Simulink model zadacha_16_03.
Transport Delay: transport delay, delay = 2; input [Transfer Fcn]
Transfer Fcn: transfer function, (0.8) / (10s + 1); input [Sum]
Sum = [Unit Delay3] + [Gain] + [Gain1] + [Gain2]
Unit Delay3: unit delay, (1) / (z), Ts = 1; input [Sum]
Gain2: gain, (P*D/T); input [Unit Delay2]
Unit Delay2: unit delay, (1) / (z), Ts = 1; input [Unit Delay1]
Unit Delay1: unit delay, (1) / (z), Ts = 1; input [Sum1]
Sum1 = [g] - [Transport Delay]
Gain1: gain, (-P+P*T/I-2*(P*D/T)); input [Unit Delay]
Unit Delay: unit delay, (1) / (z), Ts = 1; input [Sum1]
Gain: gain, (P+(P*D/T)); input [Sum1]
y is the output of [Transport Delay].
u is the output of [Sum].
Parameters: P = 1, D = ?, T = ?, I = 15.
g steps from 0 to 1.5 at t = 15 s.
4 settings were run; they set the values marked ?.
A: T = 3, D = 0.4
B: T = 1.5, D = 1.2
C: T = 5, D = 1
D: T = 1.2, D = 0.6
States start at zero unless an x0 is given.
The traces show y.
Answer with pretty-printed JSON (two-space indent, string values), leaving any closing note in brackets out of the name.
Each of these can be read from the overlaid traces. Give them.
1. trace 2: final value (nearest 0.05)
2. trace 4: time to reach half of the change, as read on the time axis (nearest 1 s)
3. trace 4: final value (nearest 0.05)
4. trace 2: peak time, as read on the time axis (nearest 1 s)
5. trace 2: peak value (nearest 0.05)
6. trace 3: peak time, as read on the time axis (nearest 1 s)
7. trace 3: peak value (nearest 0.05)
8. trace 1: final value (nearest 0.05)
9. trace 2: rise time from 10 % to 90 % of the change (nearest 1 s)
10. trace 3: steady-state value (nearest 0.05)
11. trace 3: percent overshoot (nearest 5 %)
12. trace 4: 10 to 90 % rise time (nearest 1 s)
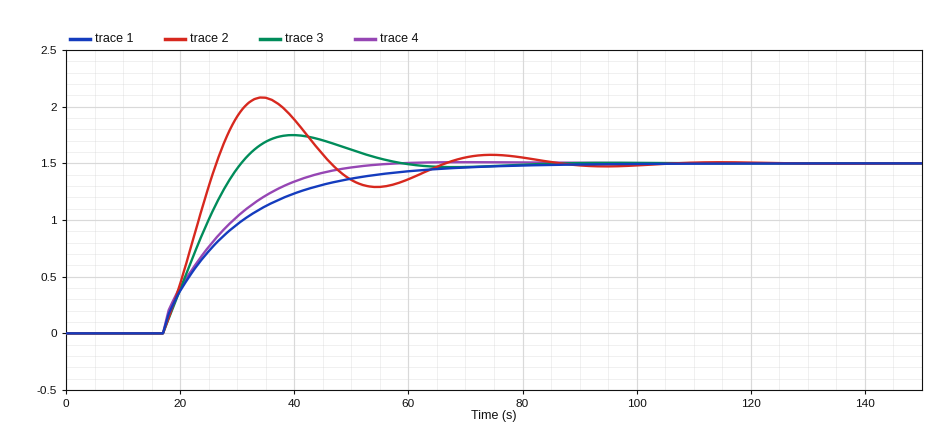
{
  "trace 2: final value": "1.50",
  "trace 4: time to reach half of the change, as read on the time axis": "25 s",
  "trace 4: final value": "1.50",
  "trace 2: peak time, as read on the time axis": "34 s",
  "trace 2: peak value": "2.10",
  "trace 3: peak time, as read on the time axis": "40 s",
  "trace 3: peak value": "1.75",
  "trace 1: final value": "1.50",
  "trace 2: rise time from 10 % to 90 % of the change": "7 s",
  "trace 3: steady-state value": "1.50",
  "trace 3: percent overshoot": "15 %",
  "trace 4: 10 to 90 % rise time": "23 s"
}
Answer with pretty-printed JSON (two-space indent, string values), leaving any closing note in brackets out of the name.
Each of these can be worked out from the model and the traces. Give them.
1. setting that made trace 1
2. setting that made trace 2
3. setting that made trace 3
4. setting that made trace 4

{
  "setting that made trace 1": "D",
  "setting that made trace 2": "C",
  "setting that made trace 3": "A",
  "setting that made trace 4": "B"
}
